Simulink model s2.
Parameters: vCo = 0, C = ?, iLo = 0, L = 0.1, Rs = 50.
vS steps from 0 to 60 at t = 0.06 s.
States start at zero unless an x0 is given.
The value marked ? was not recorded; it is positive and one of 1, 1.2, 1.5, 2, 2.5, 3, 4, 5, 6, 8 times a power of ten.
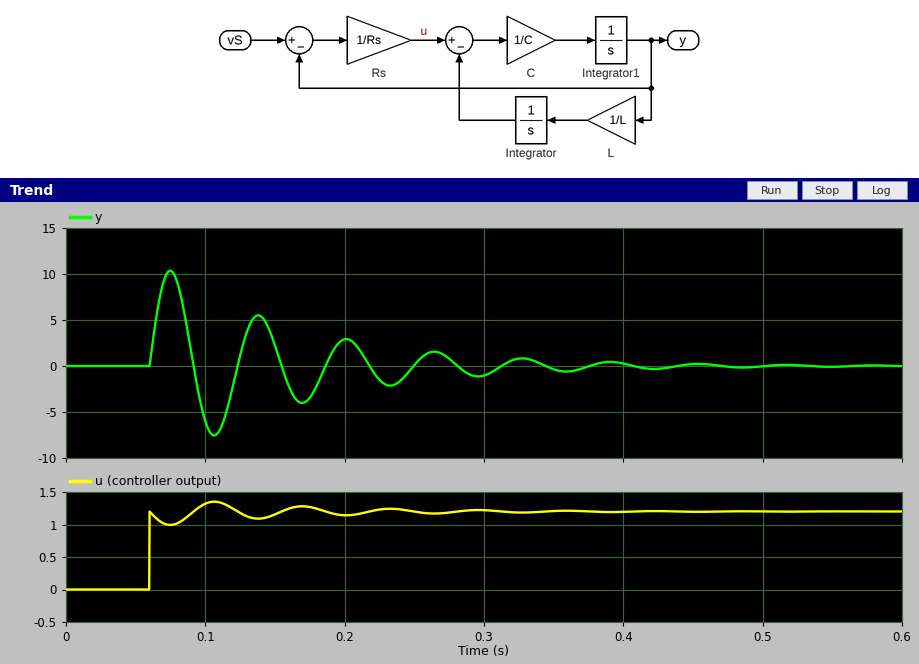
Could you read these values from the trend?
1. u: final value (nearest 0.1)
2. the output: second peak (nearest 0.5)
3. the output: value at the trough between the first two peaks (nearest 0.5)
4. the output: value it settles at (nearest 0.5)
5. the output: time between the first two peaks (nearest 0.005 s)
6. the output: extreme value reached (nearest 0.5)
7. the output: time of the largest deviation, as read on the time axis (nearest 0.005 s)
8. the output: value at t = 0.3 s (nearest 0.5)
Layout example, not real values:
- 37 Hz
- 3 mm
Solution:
- 1.2
- 5.5
- -7.5
- 0.0
- 0.065 s
- 10.5
- 0.075 s
- -1.0
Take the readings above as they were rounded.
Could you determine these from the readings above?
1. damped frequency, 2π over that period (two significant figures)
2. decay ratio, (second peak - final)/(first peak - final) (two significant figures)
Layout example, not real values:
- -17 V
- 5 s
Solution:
- 97 rad/s
- 0.52
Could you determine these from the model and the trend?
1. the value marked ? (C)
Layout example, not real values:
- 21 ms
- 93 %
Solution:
- 0.001
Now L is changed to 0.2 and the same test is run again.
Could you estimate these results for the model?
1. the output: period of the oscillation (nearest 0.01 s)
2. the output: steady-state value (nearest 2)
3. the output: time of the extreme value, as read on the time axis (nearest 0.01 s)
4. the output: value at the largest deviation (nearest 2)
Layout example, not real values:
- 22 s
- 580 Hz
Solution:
- 0.09 s
- 0
- 0.08 s
- 14
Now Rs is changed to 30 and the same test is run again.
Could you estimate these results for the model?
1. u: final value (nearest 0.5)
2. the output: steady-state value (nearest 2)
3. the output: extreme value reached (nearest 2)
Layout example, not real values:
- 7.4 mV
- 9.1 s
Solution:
- 2.0
- 0
- 16
